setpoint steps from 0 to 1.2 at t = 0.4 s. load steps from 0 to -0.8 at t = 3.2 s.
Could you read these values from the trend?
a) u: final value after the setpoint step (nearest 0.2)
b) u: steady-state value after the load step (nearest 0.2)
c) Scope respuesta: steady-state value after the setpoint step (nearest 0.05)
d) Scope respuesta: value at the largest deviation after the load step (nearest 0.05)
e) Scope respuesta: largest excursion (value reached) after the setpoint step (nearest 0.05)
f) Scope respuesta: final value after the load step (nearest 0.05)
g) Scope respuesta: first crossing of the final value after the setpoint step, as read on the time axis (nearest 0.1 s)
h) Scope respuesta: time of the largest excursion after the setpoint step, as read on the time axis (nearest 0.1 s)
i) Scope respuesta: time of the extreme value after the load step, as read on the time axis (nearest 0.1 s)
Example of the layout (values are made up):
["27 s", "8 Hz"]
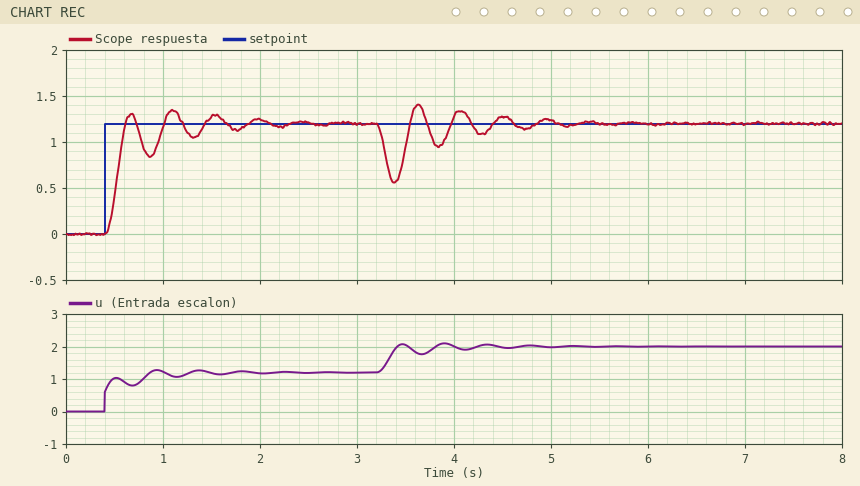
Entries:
["1.2", "2.0", "1.20", "0.55", "1.35", "1.20", "0.6 s", "1.1 s", "3.4 s"]
